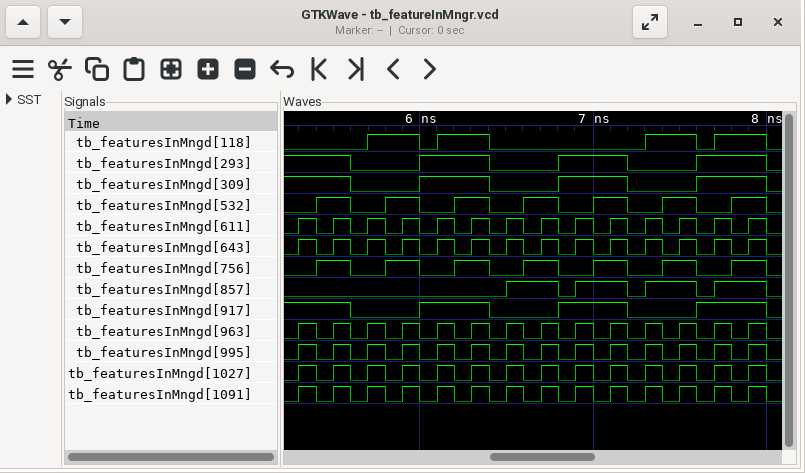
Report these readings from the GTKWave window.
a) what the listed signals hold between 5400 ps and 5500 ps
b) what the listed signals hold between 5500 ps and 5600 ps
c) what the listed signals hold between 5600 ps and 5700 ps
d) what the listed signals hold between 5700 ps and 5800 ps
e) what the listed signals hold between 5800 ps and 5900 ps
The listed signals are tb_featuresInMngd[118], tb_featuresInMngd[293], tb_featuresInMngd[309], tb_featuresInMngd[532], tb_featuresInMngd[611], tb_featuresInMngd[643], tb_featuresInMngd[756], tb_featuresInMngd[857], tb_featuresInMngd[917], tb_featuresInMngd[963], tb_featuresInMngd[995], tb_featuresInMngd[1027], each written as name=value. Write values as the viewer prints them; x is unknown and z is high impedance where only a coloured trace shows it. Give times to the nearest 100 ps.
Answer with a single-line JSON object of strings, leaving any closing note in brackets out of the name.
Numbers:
{"what the listed signals hold between 5400 ps and 5500 ps": "tb_featuresInMngd[118]=0, tb_featuresInMngd[293]=1, tb_featuresInMngd[309]=1, tb_featuresInMngd[532]=1, tb_featuresInMngd[611]=0, tb_featuresInMngd[643]=0, tb_featuresInMngd[756]=1, tb_featuresInMngd[857]=0, tb_featuresInMngd[917]=1, tb_featuresInMngd[963]=0, tb_featuresInMngd[995]=0, tb_featuresInMngd[1027]=0", "what the listed signals hold between 5500 ps and 5600 ps": "tb_featuresInMngd[118]=0, tb_featuresInMngd[293]=1, tb_featuresInMngd[309]=1, tb_featuresInMngd[532]=1, tb_featuresInMngd[611]=1, tb_featuresInMngd[643]=1, tb_featuresInMngd[756]=1, tb_featuresInMngd[857]=0, tb_featuresInMngd[917]=1, tb_featuresInMngd[963]=1, tb_featuresInMngd[995]=1, tb_featuresInMngd[1027]=1", "what the listed signals hold between 5600 ps and 5700 ps": "tb_featuresInMngd[118]=0, tb_featuresInMngd[293]=0, tb_featuresInMngd[309]=0, tb_featuresInMngd[532]=0, tb_featuresInMngd[611]=0, tb_featuresInMngd[643]=0, tb_featuresInMngd[756]=0, tb_featuresInMngd[857]=0, tb_featuresInMngd[917]=0, tb_featuresInMngd[963]=0, tb_featuresInMngd[995]=0, tb_featuresInMngd[1027]=0", "what the listed signals hold between 5700 ps and 5800 ps": "tb_featuresInMngd[118]=1, tb_featuresInMngd[293]=0, tb_featuresInMngd[309]=0, tb_featuresInMngd[532]=0, tb_featuresInMngd[611]=1, tb_featuresInMngd[643]=1, tb_featuresInMngd[756]=0, tb_featuresInMngd[857]=0, tb_featuresInMngd[917]=0, tb_featuresInMngd[963]=1, tb_featuresInMngd[995]=1, tb_featuresInMngd[1027]=1", "what the listed signals hold between 5800 ps and 5900 ps": "tb_featuresInMngd[118]=1, tb_featuresInMngd[293]=0, tb_featuresInMngd[309]=0, tb_featuresInMngd[532]=1, tb_featuresInMngd[611]=0, tb_featuresInMngd[643]=0, tb_featuresInMngd[756]=1, tb_featuresInMngd[857]=0, tb_featuresInMngd[917]=0, tb_featuresInMngd[963]=0, tb_featuresInMngd[995]=0, tb_featuresInMngd[1027]=0"}
